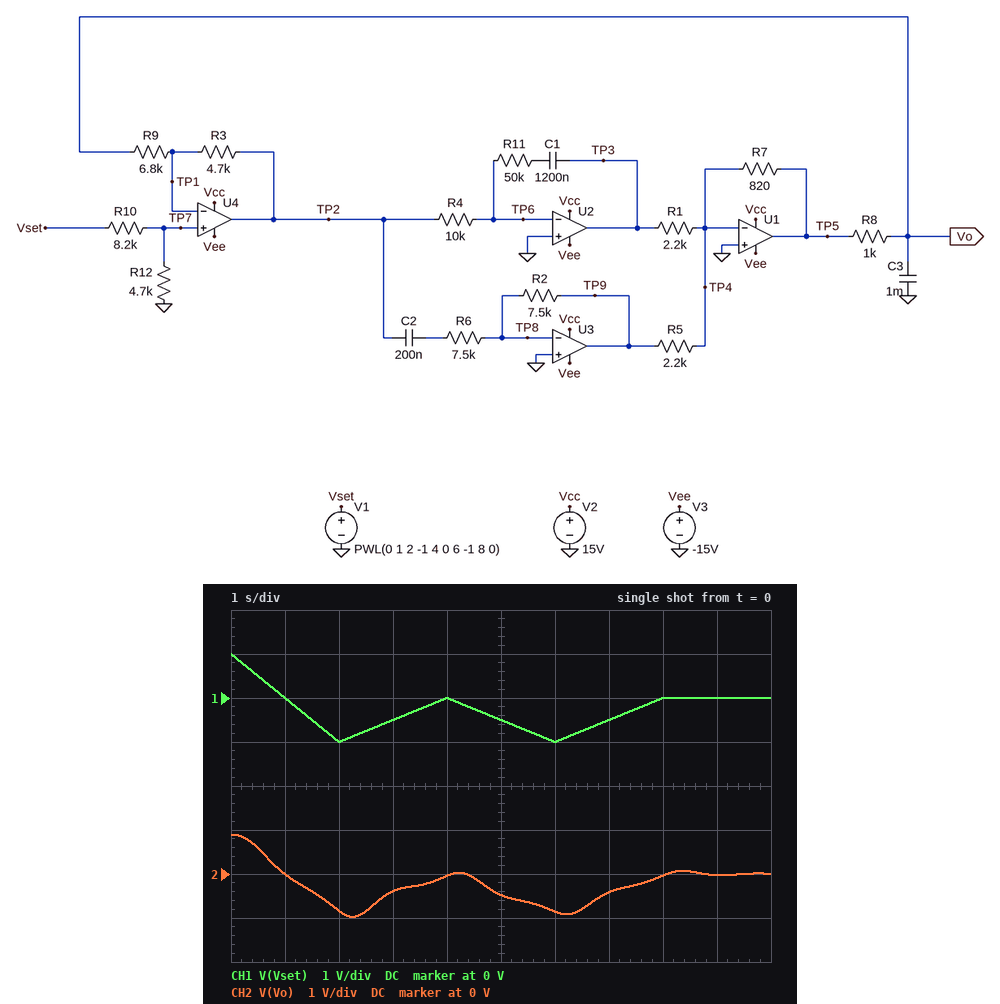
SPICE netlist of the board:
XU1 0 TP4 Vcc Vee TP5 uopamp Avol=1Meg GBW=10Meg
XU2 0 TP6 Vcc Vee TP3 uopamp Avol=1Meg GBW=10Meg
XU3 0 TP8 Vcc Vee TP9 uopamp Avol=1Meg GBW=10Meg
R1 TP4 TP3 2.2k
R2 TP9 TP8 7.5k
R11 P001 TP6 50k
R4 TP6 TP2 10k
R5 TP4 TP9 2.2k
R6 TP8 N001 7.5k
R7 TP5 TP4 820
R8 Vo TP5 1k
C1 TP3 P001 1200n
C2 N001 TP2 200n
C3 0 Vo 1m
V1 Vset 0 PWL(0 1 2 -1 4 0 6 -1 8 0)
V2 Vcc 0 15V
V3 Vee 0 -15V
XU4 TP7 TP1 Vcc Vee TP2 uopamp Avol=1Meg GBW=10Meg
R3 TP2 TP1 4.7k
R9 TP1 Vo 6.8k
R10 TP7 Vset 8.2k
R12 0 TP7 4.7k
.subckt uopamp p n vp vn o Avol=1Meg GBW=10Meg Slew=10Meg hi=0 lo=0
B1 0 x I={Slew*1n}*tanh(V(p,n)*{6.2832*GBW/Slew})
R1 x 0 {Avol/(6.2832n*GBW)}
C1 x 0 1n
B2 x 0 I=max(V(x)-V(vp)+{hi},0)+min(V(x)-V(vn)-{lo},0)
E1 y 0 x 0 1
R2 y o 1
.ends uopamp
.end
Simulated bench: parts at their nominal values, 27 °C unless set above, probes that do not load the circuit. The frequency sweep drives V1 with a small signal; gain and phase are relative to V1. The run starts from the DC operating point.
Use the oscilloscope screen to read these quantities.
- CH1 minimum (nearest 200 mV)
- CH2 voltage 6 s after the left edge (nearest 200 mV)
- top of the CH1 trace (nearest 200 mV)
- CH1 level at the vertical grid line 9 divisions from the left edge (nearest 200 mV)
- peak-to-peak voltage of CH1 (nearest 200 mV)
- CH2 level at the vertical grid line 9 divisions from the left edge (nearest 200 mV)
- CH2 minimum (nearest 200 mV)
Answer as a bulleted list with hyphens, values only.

- -1.0 V
- -800 mV
- 1.0 V
- 0 V
- 2.0 V
- 0 V
- -1.0 V
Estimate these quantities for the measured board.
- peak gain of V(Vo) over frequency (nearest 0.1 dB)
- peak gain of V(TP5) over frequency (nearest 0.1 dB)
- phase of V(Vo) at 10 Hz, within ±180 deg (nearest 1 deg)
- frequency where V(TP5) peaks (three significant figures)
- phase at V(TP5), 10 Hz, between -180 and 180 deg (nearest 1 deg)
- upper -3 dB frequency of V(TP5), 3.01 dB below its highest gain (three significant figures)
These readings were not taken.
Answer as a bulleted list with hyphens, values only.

- 5.2 dB
- 18.5 dB
- -101 deg
- 738 mHz
- -13 deg
- 963 mHz
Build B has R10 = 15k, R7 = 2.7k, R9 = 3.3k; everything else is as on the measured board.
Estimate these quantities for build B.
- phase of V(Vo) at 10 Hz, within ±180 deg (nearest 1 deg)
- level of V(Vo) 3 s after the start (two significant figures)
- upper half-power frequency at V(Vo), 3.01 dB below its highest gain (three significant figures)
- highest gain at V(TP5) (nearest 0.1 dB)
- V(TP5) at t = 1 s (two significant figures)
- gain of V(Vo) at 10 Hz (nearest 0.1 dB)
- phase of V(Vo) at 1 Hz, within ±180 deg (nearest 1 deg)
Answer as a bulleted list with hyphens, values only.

- -94 deg
- -200 mV
- 2.46 Hz
- 17.3 dB
- -400 mV
- -24.3 dB
- -10 deg
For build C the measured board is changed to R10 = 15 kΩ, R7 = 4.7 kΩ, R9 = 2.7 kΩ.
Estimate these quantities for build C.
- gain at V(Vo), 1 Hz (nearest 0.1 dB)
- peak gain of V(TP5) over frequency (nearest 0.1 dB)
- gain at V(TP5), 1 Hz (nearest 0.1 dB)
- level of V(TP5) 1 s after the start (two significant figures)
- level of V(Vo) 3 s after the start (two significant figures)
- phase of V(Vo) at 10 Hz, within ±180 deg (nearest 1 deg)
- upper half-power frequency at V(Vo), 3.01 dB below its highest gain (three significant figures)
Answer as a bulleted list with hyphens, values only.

- -7.6 dB
- 19.0 dB
- 8.5 dB
- -370 mV
- -190 mV
- -85 deg
- 3.96 Hz
